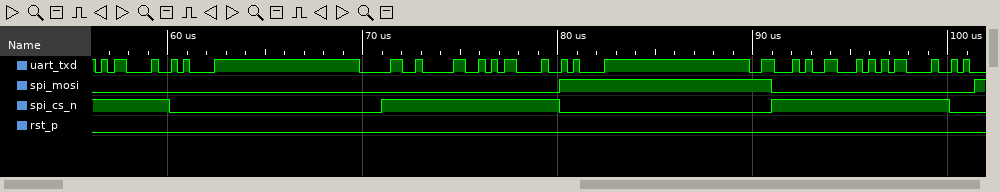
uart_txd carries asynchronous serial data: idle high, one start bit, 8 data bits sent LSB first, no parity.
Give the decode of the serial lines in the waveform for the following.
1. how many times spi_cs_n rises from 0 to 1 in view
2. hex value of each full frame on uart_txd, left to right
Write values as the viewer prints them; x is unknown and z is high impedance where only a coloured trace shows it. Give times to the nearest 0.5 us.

2
0D, 0A, 30, 30, 0D, 0A, 46, 46, 0D
